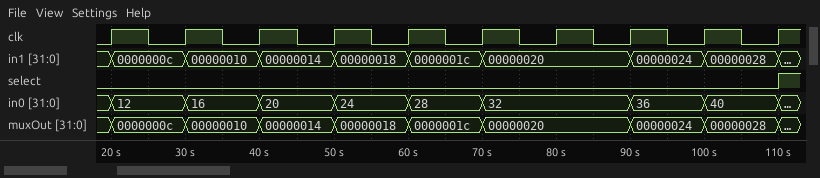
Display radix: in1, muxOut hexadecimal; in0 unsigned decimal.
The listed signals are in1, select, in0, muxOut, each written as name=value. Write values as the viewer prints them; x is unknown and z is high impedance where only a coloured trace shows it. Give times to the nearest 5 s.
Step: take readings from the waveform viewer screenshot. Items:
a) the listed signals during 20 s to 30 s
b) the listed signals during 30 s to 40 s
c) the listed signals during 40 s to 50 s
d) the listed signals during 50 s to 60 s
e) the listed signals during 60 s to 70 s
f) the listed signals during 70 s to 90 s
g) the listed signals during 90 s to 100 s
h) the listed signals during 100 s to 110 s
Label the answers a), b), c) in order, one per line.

a) in1=0000000c, select=0, in0=12, muxOut=0000000c
b) in1=00000010, select=0, in0=16, muxOut=00000010
c) in1=00000014, select=0, in0=20, muxOut=00000014
d) in1=00000018, select=0, in0=24, muxOut=00000018
e) in1=0000001c, select=0, in0=28, muxOut=0000001c
f) in1=00000020, select=0, in0=32, muxOut=00000020
g) in1=00000024, select=0, in0=36, muxOut=00000024
h) in1=00000028, select=0, in0=40, muxOut=00000028
